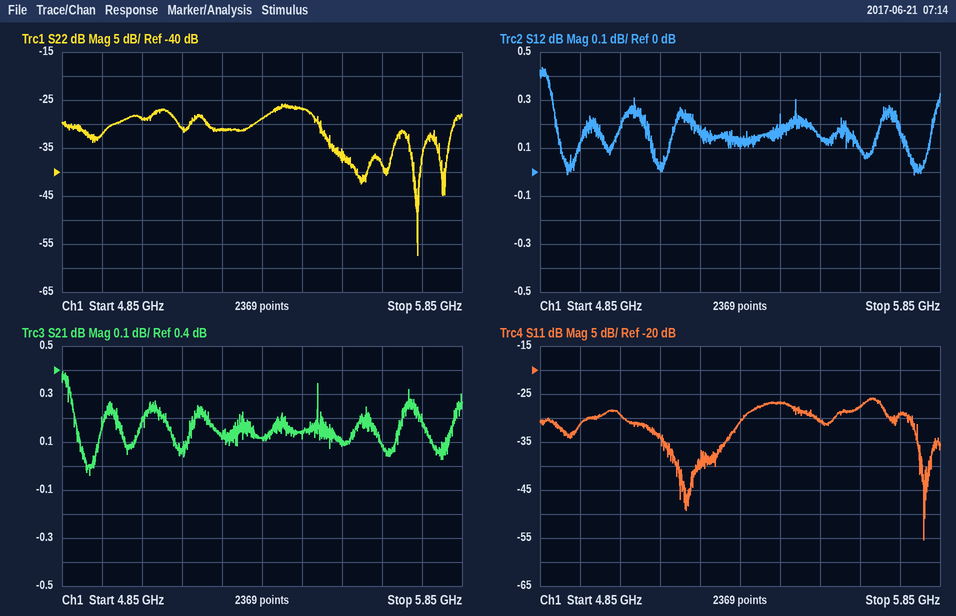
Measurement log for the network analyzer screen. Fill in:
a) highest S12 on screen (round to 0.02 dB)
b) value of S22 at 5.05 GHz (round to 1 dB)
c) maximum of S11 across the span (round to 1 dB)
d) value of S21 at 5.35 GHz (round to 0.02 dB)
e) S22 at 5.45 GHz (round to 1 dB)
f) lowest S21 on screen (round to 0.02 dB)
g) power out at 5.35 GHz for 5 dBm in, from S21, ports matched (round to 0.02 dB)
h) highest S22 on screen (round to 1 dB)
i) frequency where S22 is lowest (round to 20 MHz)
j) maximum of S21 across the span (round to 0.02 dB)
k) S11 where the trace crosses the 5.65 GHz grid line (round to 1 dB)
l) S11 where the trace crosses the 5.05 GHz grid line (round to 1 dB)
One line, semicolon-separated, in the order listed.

0.44 dB; -29 dB; -26 dB; 0.12 dB; -27 dB; -0.04 dB; 5.12 dBm; -26 dB; 5.74 GHz; 0.40 dB; -28 dB; -29 dB
